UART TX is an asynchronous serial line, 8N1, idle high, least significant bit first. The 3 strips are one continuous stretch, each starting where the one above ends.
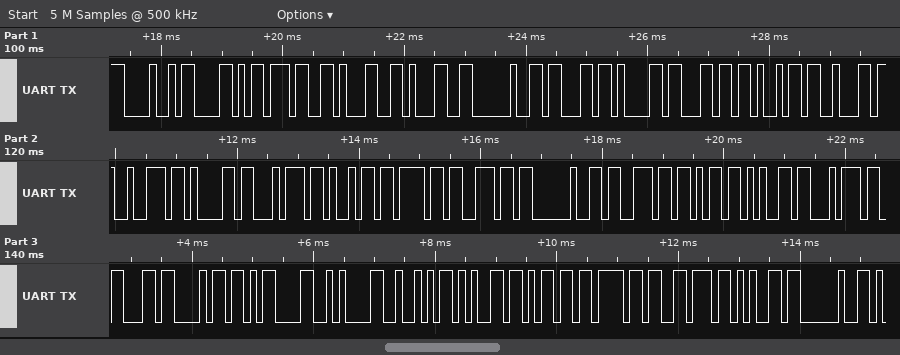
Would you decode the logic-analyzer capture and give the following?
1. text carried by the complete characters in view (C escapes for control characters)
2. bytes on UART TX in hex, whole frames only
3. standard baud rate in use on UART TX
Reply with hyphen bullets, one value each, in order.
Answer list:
- "HX711 calibration sketch\r\nRemove "
- 48 58 37 31 31 20 63 61 6C 69 62 72 61 74 69 6F 6E 20 73 6B 65 74 63 68 0D 0A 52 65 6D 6F 76 65 20
- 9600 baud
